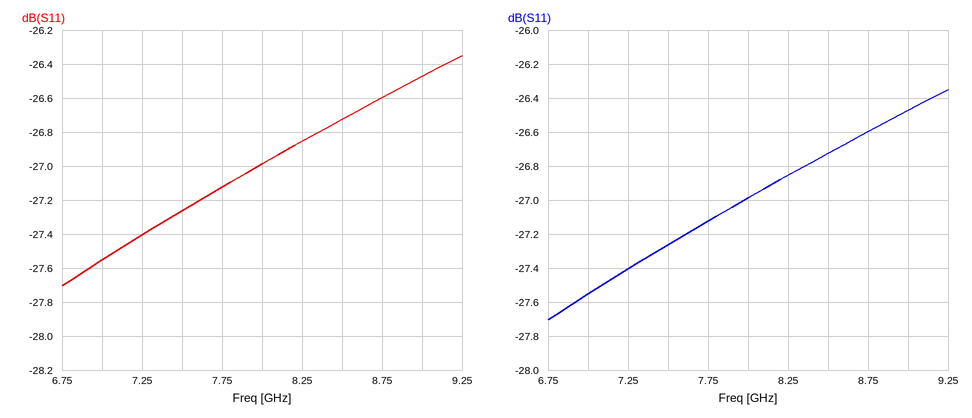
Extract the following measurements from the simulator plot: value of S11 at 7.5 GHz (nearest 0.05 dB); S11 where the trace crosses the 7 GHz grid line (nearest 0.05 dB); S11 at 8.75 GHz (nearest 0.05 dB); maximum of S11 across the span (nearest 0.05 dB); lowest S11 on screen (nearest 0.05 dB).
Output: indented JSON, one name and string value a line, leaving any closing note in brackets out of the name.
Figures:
{
  "value of S11 at 7.5 GHz": "-27.25 dB",
  "S11 where the trace crosses the 7 GHz grid line": "-27.55 dB",
  "S11 at 8.75 GHz": "-26.60 dB",
  "maximum of S11 across the span": "-26.35 dB",
  "lowest S11 on screen": "-27.70 dB"
}
